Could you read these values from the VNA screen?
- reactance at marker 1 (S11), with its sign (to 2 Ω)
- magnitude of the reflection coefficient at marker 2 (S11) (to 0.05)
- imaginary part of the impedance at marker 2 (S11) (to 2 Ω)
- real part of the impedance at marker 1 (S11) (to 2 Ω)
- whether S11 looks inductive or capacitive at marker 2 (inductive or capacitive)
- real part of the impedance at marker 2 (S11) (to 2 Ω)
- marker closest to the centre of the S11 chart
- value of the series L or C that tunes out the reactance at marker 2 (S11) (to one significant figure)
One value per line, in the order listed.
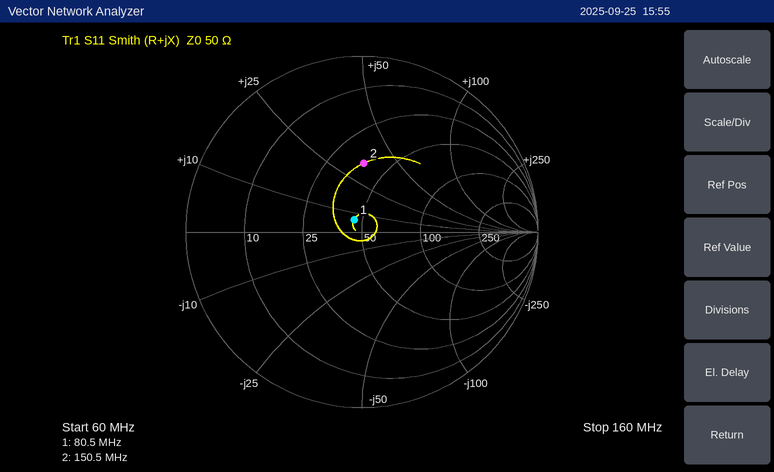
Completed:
+6 Ω
0.40
+34 Ω
46 Ω
inductive
38 Ω
marker 1
30 pF
